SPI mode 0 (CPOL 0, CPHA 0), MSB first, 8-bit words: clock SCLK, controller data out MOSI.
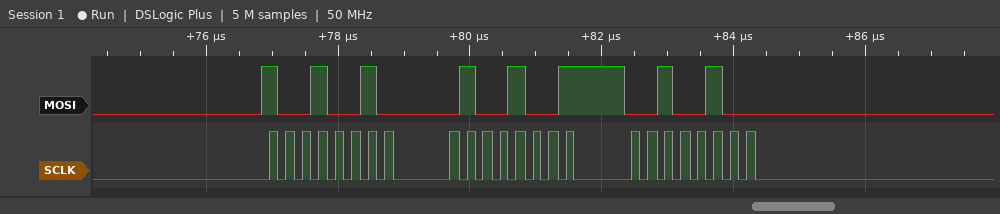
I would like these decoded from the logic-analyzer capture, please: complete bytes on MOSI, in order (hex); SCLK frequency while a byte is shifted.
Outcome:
0x92 0x49 0x24
4 MHz
